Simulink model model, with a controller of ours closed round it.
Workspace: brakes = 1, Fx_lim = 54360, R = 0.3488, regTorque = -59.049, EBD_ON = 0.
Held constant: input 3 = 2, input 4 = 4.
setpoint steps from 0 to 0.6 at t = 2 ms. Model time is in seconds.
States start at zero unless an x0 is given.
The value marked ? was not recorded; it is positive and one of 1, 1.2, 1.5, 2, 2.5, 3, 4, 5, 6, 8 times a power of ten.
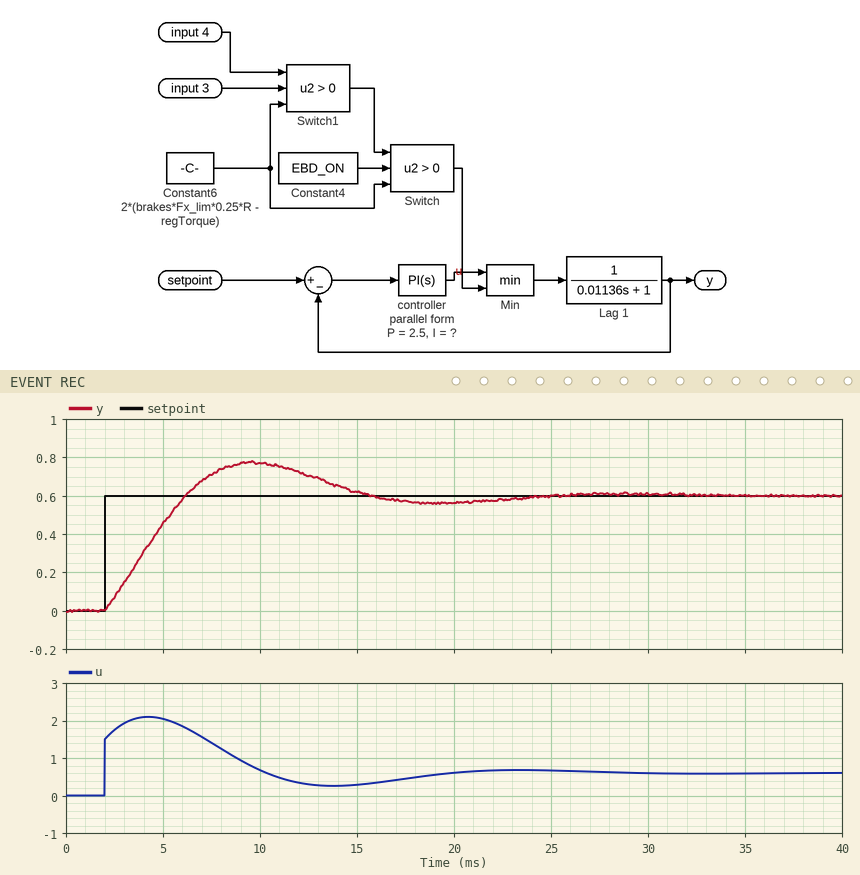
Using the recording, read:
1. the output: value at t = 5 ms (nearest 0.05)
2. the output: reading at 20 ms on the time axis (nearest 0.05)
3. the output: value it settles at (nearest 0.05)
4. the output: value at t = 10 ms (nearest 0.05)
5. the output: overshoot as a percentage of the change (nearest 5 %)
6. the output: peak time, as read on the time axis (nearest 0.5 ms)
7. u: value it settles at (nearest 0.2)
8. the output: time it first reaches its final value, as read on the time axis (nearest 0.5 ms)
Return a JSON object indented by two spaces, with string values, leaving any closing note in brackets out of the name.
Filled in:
{
  "the output: value at t = 5 ms": "0.45",
  "the output: reading at 20 ms on the time axis": "0.55",
  "the output: value it settles at": "0.60",
  "the output: value at t = 10 ms": "0.75",
  "the output: overshoot as a percentage of the change": "30 %",
  "the output: peak time, as read on the time axis": "9.5 ms",
  "u: value it settles at": "0.6",
  "the output: time it first reaches its final value, as read on the time axis": "6.0 ms"
}
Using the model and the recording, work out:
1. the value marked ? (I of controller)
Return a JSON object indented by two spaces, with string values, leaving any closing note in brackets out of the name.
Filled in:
{
  "the value marked ?": "1500"
}
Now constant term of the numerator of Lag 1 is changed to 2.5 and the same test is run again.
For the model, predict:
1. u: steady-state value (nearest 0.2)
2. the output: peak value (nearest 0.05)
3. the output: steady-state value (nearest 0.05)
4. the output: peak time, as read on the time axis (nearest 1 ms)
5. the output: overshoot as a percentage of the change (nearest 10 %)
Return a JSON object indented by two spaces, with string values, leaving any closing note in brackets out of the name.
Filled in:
{
  "u: steady-state value": "0.2",
  "the output: peak value": "0.75",
  "the output: steady-state value": "0.60",
  "the output: peak time, as read on the time axis": "6 ms",
  "the output: overshoot as a percentage of the change": "20 %"
}
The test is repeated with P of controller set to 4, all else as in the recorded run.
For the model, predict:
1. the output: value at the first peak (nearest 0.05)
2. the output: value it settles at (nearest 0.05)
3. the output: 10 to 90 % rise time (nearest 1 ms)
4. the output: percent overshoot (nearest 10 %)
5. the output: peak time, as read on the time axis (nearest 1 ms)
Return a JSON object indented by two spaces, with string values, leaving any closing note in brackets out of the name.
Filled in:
{
  "the output: value at the first peak": "0.70",
  "the output: value it settles at": "0.60",
  "the output: 10 to 90 % rise time": "3 ms",
  "the output: percent overshoot": "20 %",
  "the output: peak time, as read on the time axis": "9 ms"
}
